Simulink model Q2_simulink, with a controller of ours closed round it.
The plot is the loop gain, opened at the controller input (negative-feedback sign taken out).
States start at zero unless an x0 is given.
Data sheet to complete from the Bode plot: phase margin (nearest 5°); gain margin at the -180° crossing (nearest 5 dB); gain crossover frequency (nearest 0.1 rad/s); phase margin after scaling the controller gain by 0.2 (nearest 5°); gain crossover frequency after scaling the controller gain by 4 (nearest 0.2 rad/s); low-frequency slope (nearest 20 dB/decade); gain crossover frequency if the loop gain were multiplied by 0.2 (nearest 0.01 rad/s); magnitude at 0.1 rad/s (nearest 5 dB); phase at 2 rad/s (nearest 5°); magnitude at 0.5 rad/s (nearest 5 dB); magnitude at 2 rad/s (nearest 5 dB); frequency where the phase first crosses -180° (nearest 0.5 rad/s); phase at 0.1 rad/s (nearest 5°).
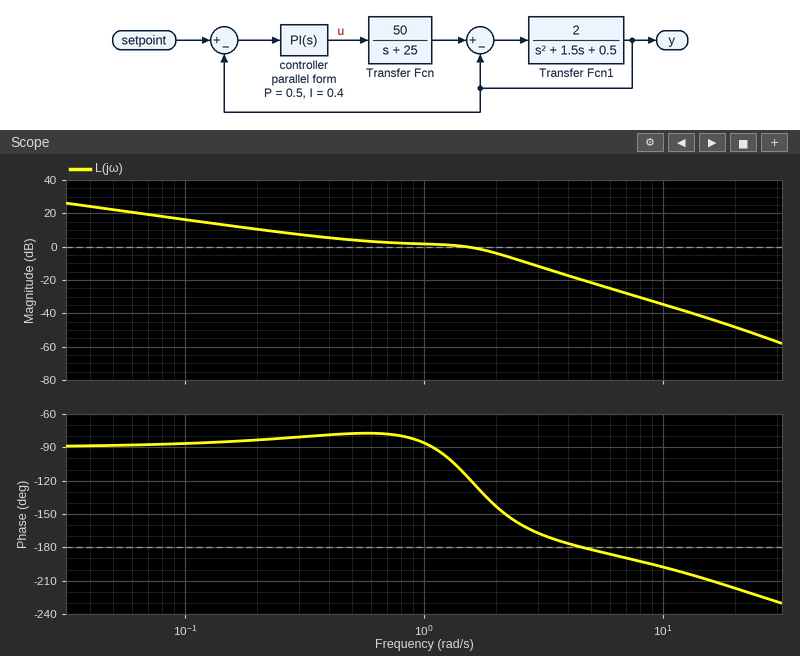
65°
20 dB
1.5 rad/s
95°
3.0 rad/s
-20 dB/decade
0.13 rad/s
15 dB
-145°
5 dB
-5 dB
4.5 rad/s
-85°
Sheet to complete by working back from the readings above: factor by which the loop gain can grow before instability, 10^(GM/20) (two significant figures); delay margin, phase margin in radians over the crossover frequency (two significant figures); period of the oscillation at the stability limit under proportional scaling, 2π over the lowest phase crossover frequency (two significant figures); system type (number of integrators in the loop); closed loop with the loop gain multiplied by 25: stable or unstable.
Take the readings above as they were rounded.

10
0.76 s
1.4 s
1
unstable
